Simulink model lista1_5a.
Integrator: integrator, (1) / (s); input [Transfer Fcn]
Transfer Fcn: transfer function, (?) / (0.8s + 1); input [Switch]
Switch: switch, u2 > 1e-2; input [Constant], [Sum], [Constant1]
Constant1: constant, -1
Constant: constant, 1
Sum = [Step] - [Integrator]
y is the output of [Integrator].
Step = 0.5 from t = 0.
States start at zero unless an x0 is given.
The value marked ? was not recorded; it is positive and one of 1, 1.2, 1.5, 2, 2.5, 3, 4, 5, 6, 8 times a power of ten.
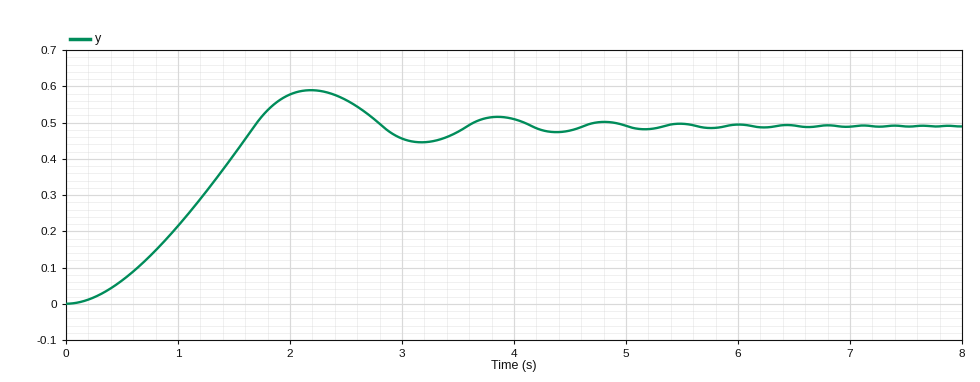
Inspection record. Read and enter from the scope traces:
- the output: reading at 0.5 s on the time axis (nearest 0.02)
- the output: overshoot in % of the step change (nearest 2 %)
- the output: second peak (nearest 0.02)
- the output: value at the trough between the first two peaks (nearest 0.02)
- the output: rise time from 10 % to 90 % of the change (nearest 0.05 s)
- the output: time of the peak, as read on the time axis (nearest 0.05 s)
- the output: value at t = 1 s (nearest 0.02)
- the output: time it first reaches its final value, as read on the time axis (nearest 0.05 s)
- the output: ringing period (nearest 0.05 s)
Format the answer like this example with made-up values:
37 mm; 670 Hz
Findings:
0.06; 20 %; 0.52; 0.44; 1.15 s; 2.20 s; 0.22; 1.70 s; 1.65 s
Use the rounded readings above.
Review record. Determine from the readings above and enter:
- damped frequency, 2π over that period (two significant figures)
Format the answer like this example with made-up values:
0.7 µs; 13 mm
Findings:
3.8 rad/s
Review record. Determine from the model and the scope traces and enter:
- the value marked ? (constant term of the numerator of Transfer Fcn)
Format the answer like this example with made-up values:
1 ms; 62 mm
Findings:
0.5
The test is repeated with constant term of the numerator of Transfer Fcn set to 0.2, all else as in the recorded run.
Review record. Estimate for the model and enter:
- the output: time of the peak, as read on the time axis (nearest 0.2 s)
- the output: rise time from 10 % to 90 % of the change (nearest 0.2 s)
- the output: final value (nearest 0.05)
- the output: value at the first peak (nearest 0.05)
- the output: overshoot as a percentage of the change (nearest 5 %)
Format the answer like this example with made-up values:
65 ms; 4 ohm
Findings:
3.8 s; 2.2 s; 0.50; 0.55; 10 %
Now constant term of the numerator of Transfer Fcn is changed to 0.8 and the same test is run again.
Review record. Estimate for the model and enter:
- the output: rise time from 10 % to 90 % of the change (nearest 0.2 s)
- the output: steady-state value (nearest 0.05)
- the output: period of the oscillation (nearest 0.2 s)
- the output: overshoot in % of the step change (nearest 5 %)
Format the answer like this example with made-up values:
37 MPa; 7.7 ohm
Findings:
0.8 s; 0.50; 1.6 s; 25 %
